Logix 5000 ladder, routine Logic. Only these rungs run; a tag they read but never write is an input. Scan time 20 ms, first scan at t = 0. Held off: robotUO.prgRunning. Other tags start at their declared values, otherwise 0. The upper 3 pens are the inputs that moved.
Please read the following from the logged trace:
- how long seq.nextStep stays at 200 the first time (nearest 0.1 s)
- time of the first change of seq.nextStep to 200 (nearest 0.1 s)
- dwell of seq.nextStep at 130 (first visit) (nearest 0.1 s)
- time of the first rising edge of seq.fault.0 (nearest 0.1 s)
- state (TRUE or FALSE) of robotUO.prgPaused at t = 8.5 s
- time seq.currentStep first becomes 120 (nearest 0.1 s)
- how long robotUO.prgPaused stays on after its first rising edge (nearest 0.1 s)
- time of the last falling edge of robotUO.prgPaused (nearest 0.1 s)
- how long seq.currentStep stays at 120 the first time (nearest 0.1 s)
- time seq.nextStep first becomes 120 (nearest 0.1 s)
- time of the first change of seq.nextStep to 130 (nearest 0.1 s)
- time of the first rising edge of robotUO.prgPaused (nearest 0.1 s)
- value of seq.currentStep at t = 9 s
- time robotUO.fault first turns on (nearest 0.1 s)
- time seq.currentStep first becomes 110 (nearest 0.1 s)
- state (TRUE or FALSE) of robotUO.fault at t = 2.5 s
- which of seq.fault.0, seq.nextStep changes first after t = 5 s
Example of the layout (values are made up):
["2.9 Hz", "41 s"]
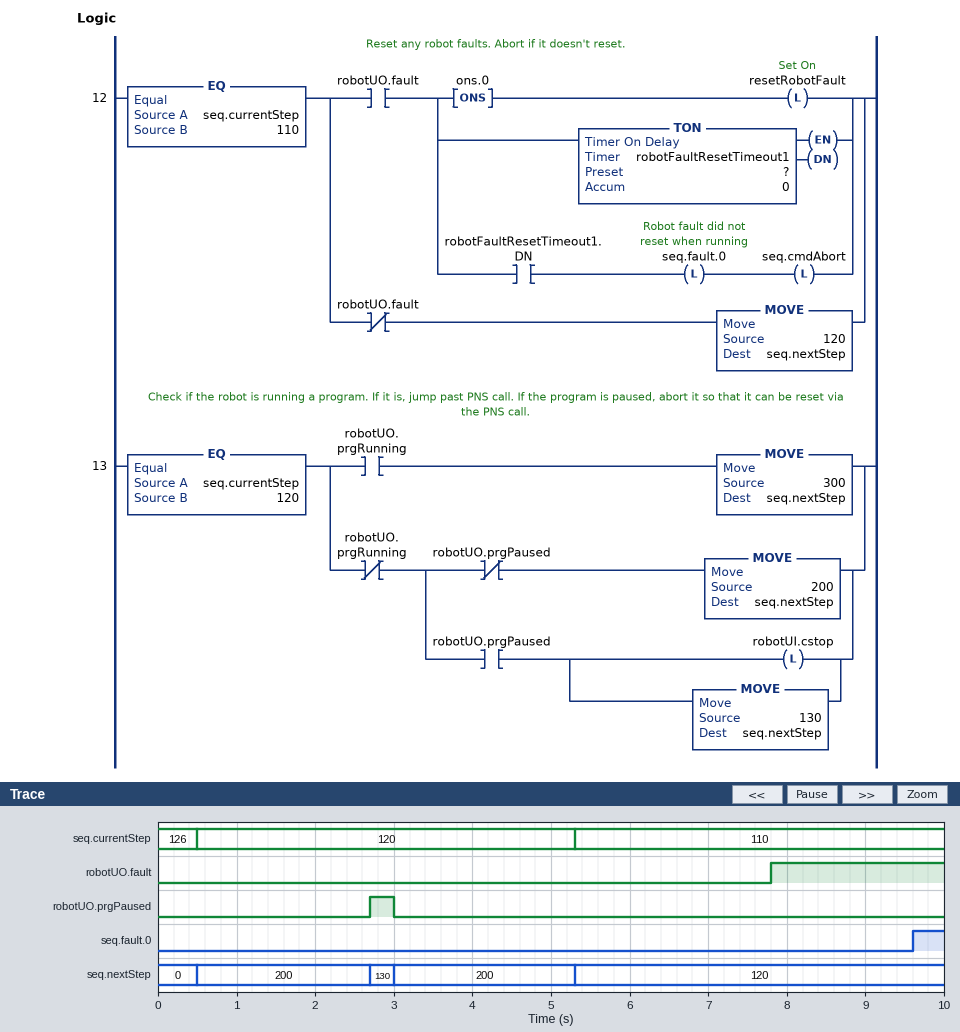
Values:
["2.2 s", "0.5 s", "0.3 s", "9.6 s", "FALSE", "0.5 s", "0.3 s", "3.0 s", "4.8 s", "5.3 s", "2.7 s", "2.7 s", "110", "7.8 s", "5.3 s", "FALSE", "seq.nextStep"]
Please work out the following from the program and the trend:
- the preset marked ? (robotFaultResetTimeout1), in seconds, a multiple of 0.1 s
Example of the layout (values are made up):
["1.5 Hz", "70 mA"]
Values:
["1.8 s"]
